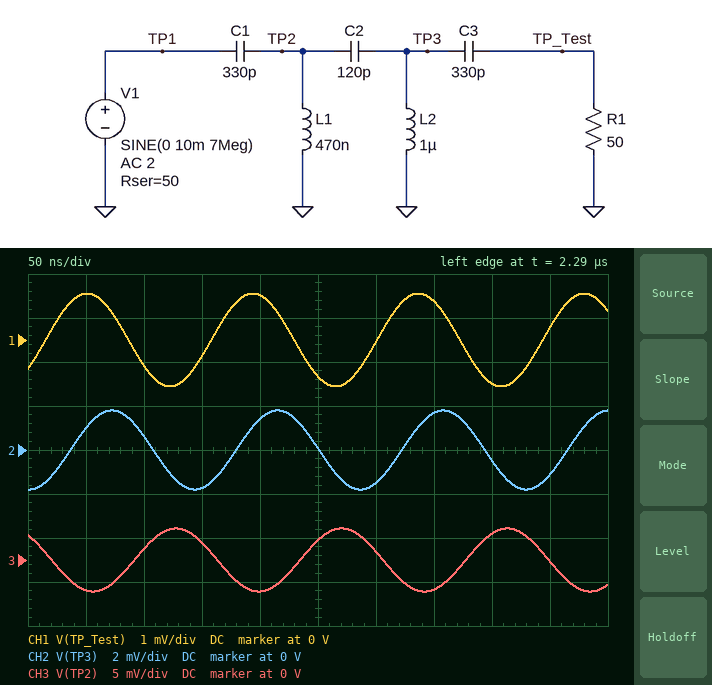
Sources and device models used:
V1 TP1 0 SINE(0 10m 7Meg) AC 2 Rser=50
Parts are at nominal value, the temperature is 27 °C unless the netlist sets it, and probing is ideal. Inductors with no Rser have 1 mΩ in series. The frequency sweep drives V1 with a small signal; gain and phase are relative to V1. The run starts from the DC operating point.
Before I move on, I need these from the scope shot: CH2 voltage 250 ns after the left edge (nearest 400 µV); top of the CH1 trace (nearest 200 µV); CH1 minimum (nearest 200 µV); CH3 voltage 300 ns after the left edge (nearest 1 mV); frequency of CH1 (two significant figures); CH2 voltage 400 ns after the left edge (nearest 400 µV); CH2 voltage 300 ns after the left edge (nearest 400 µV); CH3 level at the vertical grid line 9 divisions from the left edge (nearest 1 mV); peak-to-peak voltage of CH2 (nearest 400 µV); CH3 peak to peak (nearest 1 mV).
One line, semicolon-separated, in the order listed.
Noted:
0 V; 1.0 mV; -1.0 mV; 1 mV; 7.0 MHz; -400 µV; -1.6 mV; 0 V; 3.6 mV; 7 mV
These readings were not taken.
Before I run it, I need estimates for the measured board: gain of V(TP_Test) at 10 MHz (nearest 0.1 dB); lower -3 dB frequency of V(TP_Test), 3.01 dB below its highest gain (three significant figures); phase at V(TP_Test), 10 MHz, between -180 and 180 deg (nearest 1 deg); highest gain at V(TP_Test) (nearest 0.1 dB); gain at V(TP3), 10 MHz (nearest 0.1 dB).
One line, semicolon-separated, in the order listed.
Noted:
-9.9 dB; 10.9 MHz; -143 deg; -6.0 dB; -7.0 dB
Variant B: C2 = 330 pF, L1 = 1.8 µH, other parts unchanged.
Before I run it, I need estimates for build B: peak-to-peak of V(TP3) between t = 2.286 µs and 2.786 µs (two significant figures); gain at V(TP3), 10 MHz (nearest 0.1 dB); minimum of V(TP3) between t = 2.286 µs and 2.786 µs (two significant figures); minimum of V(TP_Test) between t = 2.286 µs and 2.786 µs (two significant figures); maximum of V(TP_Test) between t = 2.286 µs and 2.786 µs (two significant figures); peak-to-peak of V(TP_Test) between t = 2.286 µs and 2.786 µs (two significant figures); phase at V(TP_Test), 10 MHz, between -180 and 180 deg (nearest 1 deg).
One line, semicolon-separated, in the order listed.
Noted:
13 mV; -3.3 dB; -6.6 mV; -3.9 mV; 3.9 mV; 7.7 mV; 117 deg
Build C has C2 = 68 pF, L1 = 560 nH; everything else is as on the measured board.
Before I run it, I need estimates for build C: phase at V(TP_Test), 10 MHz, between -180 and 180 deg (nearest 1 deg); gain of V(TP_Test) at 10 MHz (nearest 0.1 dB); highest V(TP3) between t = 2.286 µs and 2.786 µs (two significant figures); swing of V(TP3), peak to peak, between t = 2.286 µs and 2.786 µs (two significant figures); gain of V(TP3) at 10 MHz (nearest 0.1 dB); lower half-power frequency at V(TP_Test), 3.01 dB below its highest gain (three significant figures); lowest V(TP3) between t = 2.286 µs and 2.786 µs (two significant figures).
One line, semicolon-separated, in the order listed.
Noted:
-124 deg; -12.8 dB; 1.0 mV; 2.0 mV; -9.9 dB; 15.3 MHz; -1.0 mV
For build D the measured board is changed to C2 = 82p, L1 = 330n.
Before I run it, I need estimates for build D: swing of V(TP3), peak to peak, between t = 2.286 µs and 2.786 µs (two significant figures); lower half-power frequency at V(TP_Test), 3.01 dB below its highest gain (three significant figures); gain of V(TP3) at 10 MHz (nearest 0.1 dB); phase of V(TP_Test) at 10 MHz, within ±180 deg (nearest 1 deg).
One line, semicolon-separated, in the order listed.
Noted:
1.3 mV; 18.0 MHz; -13.9 dB; -109 deg
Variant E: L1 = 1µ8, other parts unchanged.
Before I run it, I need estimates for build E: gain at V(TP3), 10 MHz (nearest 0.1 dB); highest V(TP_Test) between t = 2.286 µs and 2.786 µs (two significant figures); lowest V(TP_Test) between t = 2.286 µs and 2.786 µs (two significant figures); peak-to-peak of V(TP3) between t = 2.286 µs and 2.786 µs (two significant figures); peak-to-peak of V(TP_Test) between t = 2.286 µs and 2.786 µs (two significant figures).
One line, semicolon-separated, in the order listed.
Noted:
-4.6 dB; 3.6 mV; -3.6 mV; 12 mV; 7.2 mV
